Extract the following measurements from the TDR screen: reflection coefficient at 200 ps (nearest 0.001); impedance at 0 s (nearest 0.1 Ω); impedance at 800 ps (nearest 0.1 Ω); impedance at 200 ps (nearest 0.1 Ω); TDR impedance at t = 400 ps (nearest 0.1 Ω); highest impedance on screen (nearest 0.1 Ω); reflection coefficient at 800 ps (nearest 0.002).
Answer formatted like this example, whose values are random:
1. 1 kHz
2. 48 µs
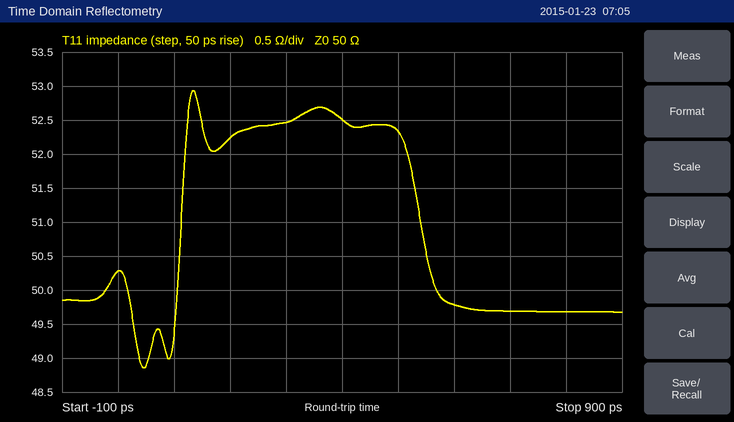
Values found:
1. +0.022
2. 50.3 Ω
3. 49.7 Ω
4. 52.2 Ω
5. 52.5 Ω
6. 52.9 Ω
7. -0.004
